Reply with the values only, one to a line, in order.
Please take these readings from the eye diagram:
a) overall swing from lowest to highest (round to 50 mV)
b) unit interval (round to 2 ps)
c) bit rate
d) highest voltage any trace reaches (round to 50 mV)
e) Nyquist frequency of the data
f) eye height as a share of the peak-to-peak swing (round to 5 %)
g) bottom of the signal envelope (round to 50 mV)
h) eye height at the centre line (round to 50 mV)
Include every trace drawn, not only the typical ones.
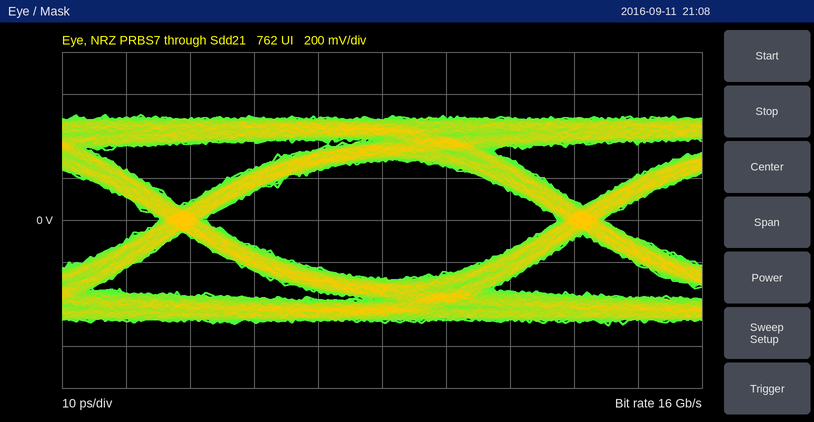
1.00 V
62 ps
16 Gb/s
500 mV
8 GHz
55 %
-500 mV
550 mV
